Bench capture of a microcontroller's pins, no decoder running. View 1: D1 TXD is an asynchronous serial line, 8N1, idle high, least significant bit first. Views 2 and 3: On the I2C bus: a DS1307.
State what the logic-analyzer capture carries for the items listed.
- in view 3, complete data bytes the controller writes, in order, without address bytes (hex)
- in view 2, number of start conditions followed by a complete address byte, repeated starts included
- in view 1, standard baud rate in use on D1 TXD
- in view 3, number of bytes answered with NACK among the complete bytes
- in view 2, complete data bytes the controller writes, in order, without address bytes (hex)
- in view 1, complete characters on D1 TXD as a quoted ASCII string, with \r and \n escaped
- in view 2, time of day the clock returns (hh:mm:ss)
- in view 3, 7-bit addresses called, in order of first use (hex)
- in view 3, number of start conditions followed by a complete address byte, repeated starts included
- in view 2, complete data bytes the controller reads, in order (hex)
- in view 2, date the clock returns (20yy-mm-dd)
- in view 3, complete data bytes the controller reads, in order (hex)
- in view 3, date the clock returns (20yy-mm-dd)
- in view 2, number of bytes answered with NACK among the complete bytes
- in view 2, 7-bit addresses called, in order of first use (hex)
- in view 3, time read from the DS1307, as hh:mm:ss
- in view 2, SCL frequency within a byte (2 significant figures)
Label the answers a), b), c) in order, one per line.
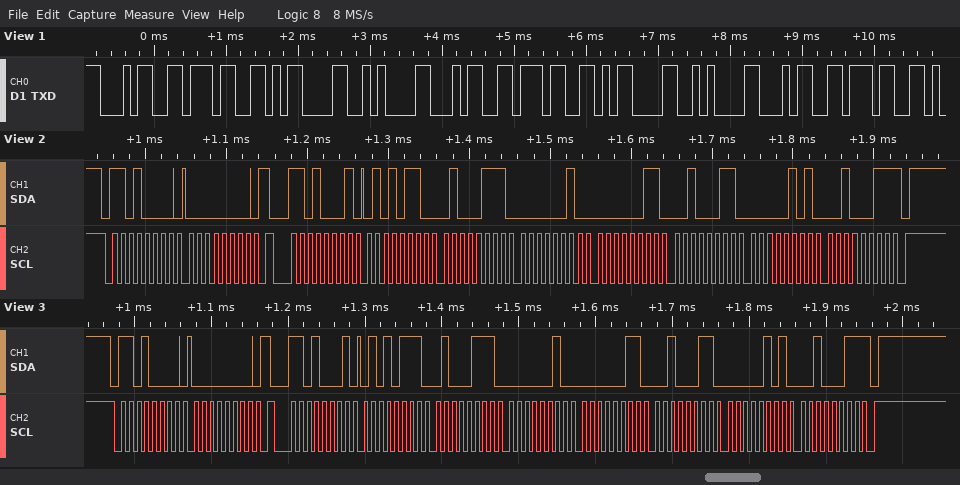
a) 00
b) 2
c) 9600 baud
d) 1
e) 00
f) "47\r\n47\r\n47"
g) 02:47:56
h) 0x68
i) 2
j) 56 47 02 03 23 05 23
k) 2023-05-23
l) 57 47 02 03 23 05 23
m) 2023-05-23
n) 1
o) 0x68
p) 02:47:57
q) 100 kHz
